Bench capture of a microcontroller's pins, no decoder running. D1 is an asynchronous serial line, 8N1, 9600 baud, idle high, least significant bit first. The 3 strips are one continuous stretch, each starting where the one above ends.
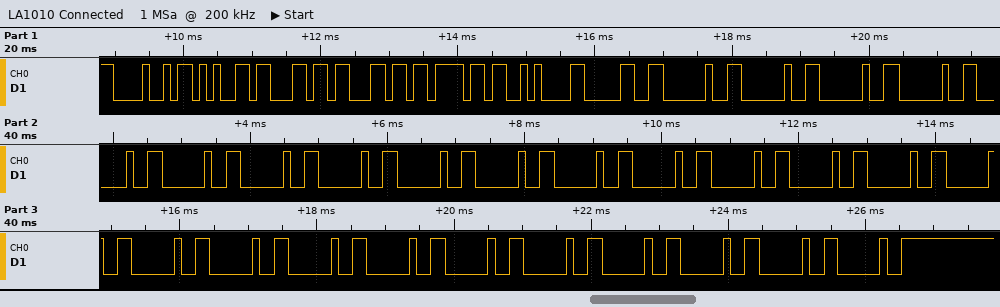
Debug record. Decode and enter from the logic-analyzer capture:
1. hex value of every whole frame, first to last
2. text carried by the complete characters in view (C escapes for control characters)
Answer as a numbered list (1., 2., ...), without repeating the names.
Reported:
1. 48 65 6C 6C 6F 0A 30 20 20 20 20 20 20 20 20 20 20 20 20 20 20 20 20 20 20 20 20 20 20 20 20 20 20
2. "Hello\n0                          "
